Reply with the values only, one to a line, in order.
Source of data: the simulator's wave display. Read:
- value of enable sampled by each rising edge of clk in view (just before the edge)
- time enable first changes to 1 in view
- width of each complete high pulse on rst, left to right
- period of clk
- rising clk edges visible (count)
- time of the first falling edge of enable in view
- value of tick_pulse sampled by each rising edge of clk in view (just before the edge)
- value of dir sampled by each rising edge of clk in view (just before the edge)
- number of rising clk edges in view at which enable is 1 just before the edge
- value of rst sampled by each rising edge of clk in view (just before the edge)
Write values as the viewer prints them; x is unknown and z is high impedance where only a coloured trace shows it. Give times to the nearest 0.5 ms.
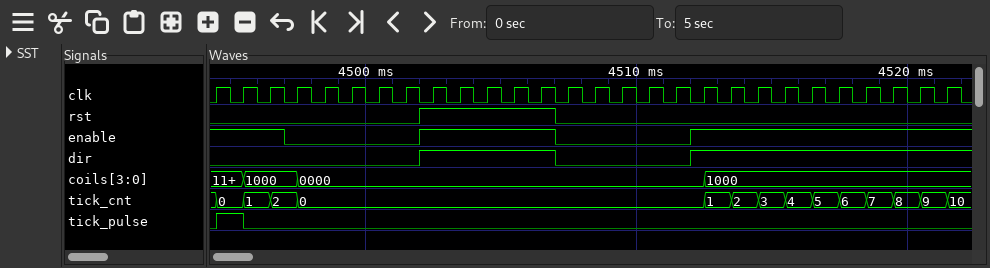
1 1 1 0 0 0 0 0 1 1 1 1 1 0 0 0 0 0 1 1 1 1 1 1 1 1 1 1
4502 ms
5 ms
1 ms
28
4497 ms
0 1 0 0 0 0 0 0 0 0 0 0 0 0 0 0 0 0 0 0 0 0 0 0 0 0 0 0
0 0 0 0 0 0 0 0 1 1 1 1 1 0 0 0 0 0 1 1 1 1 1 1 1 1 1 1
18
0 0 0 0 0 0 0 0 1 1 1 1 1 0 0 0 0 0 0 0 0 0 0 0 0 0 0 0
